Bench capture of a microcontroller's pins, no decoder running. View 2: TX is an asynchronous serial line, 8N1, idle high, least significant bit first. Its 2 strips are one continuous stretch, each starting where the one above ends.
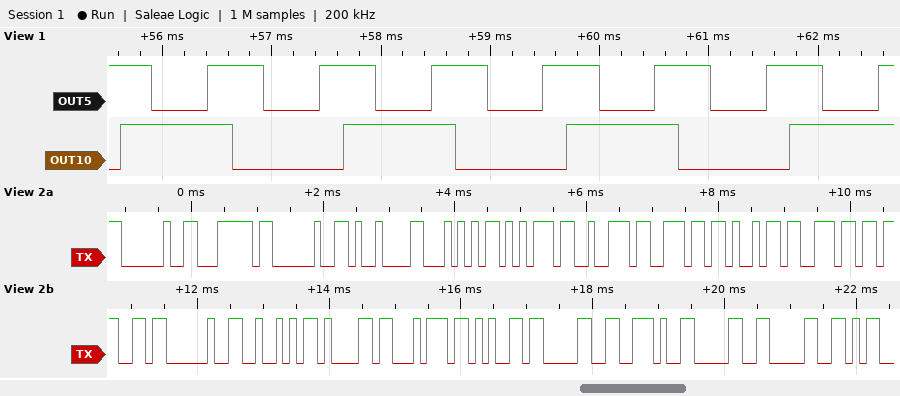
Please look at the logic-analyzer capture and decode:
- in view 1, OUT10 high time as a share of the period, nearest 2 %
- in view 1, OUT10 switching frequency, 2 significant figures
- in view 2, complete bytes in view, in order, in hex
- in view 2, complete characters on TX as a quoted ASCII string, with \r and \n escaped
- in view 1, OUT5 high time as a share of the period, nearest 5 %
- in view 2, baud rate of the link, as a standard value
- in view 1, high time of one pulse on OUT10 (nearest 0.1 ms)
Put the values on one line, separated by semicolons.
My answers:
50 %; 490 Hz; 0x20 0x7C 0x20 0x09 0x54 0x75 0x72 0x6E 0x69 0x6E 0x67 0x20 0x52 0x61 0x74 0x65 0x30 0x2E 0x30 0x30; " | \tTurning Rate0.00"; 50 %; 9600 baud; 1.0 ms
